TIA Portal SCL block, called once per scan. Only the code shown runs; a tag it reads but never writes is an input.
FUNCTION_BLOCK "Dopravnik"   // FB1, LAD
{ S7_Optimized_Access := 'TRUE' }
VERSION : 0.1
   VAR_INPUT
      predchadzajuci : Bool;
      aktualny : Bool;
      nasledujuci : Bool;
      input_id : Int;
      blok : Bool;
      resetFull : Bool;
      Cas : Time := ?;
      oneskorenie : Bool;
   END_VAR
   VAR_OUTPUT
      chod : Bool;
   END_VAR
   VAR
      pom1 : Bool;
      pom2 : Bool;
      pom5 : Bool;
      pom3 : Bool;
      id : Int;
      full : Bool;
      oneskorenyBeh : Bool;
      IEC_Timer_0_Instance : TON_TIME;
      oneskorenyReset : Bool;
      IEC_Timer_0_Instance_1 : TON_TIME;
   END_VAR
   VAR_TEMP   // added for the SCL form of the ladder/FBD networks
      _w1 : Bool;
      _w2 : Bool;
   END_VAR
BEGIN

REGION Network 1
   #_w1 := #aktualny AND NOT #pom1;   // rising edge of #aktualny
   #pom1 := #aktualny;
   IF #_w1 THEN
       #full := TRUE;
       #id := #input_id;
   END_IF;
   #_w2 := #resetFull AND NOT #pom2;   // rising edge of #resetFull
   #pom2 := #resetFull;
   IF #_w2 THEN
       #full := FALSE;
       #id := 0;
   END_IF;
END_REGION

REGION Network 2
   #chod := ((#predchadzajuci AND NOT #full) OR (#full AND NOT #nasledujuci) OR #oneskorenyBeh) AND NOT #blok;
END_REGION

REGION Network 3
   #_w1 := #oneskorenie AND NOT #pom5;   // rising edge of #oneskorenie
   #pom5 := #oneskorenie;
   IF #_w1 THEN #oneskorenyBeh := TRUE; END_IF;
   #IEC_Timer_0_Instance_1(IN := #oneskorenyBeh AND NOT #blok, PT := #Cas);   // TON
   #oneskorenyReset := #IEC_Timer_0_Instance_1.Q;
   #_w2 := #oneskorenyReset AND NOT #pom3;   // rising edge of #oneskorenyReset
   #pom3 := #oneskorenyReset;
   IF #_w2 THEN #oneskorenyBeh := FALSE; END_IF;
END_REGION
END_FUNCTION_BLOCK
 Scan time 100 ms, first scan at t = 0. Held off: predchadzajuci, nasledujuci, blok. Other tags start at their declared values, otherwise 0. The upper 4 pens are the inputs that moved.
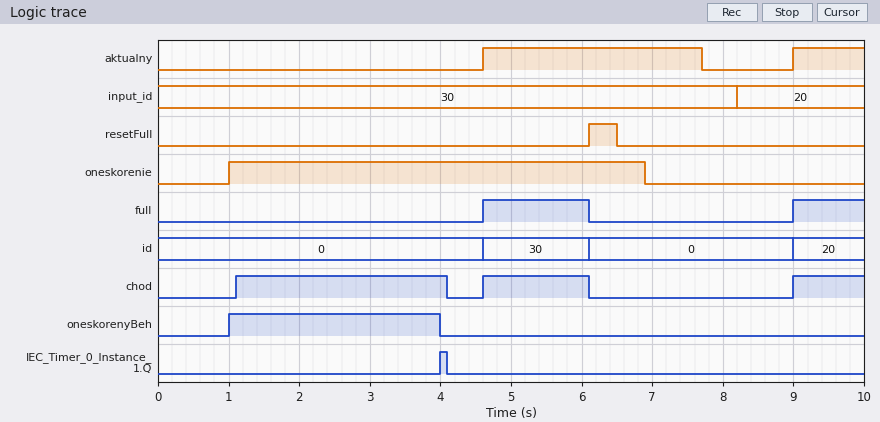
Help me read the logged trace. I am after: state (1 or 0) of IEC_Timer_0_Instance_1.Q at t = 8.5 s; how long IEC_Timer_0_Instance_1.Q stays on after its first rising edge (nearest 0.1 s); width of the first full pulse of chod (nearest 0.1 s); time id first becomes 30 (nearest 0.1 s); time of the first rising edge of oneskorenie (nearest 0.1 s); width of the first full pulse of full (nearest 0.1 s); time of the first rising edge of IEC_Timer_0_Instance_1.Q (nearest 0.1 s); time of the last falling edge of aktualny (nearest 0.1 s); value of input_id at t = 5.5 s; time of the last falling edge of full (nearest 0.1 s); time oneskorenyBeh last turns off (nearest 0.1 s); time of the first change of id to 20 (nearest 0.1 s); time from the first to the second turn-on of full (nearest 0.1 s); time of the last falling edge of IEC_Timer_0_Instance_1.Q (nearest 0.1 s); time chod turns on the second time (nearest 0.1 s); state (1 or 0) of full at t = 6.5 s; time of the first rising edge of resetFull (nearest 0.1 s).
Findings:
0
0.1 s
3.0 s
4.6 s
1.0 s
1.5 s
4.0 s
7.7 s
30
6.1 s
4.0 s
9.0 s
4.4 s
4.1 s
4.6 s
0
6.1 s
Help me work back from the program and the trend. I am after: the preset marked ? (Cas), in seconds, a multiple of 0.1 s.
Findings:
3.0 s
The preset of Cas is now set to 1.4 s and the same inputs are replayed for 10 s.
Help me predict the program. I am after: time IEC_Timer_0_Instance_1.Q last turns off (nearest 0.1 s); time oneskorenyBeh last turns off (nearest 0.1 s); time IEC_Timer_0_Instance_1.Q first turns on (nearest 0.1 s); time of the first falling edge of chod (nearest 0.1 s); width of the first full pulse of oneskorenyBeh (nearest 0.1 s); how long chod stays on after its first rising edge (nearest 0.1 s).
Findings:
2.5 s
2.4 s
2.4 s
2.5 s
1.4 s
1.4 s
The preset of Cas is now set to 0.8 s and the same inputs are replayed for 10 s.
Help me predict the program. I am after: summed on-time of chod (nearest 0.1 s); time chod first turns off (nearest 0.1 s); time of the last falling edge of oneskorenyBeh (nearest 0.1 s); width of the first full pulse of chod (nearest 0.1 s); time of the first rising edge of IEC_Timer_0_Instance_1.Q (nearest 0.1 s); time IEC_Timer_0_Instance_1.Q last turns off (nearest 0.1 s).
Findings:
3.3 s
1.9 s
1.8 s
0.8 s
1.8 s
1.9 s
